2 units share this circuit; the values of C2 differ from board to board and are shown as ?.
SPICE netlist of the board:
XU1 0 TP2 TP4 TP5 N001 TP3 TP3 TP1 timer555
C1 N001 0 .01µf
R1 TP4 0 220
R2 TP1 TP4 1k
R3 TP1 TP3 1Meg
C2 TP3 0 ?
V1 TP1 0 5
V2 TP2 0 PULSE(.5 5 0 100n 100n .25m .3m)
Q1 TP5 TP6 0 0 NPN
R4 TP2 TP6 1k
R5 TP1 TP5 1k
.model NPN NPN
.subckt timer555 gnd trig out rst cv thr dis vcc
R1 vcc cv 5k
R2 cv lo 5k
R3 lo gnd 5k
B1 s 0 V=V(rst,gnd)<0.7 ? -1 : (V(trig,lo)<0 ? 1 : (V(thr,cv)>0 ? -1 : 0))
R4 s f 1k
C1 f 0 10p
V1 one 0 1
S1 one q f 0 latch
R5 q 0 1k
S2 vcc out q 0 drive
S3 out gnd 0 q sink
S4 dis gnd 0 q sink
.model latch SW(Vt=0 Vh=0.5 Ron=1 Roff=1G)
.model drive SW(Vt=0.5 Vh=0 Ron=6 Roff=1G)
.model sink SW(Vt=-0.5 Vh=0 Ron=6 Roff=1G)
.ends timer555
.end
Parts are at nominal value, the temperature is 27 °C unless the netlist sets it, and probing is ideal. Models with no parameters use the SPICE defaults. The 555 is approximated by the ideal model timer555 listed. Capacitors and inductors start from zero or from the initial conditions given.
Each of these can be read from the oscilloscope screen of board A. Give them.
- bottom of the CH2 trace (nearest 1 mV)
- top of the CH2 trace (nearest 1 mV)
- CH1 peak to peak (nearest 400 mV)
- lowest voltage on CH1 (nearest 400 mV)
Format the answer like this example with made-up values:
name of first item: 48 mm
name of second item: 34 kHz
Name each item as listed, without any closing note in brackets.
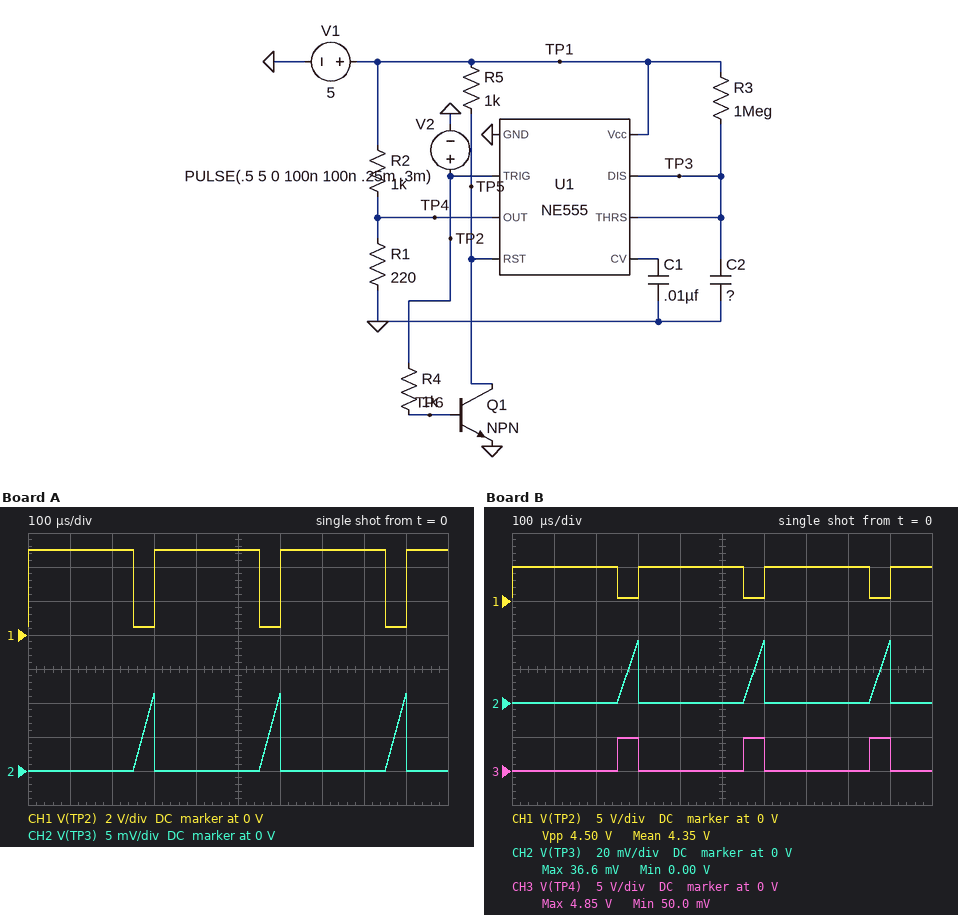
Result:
bottom of the CH2 trace: 0 V
top of the CH2 trace: 11 mV
CH1 peak to peak: 4.4 V
lowest voltage on CH1: 400 mV
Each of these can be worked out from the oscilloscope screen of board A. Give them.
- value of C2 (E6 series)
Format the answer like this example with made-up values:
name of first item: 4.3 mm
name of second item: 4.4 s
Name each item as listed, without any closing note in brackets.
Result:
value of C2: 22 nF
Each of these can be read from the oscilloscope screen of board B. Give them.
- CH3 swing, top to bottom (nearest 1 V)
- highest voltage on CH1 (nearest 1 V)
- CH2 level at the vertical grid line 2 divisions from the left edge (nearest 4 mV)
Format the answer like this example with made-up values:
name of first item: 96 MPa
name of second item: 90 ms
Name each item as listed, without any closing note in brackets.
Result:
CH3 swing, top to bottom: 5 V
highest voltage on CH1: 5 V
CH2 level at the vertical grid line 2 divisions from the left edge: 0 V
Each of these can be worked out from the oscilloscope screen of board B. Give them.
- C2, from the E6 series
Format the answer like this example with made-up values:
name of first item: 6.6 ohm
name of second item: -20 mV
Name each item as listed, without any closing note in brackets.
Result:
C2, from the E6 series: 6.8 nF
